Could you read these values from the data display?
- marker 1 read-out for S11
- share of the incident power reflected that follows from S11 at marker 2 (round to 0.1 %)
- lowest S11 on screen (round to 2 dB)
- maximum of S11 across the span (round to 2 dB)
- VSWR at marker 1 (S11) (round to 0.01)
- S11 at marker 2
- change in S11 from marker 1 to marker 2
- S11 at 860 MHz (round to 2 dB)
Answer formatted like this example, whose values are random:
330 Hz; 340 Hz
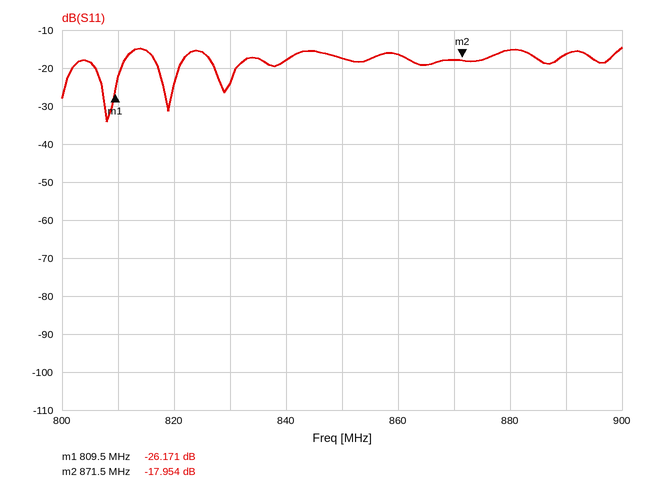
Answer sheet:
-26.171 dB; 1.6 %; -34 dB; -14 dB; 1.10; -17.954 dB; 8.217 dB; -16 dB
